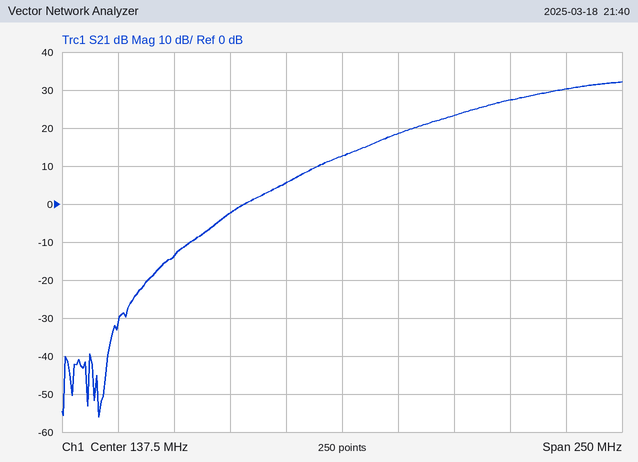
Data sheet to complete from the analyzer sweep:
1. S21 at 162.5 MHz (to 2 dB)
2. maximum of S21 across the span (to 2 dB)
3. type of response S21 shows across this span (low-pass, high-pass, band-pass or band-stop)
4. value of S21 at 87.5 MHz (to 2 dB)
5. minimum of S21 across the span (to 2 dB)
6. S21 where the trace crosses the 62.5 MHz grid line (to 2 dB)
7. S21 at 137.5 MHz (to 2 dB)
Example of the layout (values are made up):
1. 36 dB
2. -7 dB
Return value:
1. 18 dB
2. 32 dB
3. high-pass
4. -2 dB
5. -56 dB
6. -14 dB
7. 12 dB
